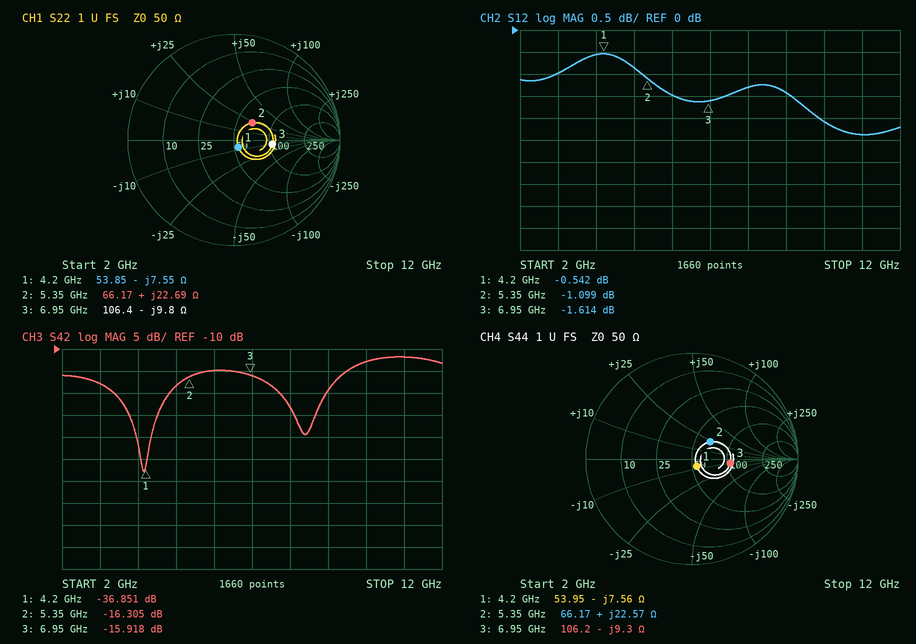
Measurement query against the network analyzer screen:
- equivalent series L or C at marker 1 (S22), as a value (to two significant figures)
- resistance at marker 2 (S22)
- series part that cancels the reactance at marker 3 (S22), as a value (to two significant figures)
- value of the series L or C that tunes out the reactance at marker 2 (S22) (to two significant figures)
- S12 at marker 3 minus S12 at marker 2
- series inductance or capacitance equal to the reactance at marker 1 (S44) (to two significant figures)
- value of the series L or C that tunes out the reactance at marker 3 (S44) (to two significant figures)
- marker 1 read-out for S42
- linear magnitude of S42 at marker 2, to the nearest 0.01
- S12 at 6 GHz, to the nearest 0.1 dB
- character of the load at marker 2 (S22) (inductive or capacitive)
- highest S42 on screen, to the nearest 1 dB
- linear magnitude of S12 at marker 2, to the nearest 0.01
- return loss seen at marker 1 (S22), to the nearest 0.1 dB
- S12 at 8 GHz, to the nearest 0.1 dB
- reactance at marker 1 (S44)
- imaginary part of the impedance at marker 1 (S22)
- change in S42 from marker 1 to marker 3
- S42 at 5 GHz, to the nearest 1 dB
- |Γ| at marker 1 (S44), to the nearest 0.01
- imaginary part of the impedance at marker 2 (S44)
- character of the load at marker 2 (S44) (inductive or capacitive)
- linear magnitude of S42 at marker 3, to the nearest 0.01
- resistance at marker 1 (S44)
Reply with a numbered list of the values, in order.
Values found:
1. 5.0 pF
2. 66.17 Ω
3. 220 pH
4. 1.3 pF
5. -0.515 dB
6. 5.0 pF
7. 210 pH
8. -36.851 dB
9. 0.15
10. -1.5 dB
11. inductive
12. -12 dB
13. 0.88
14. 21.8 dB
15. -1.3 dB
16. -7.56 Ω
17. -7.55 Ω
18. 20.933 dB
19. -18 dB
20. 0.08
21. +22.57 Ω
22. inductive
23. 0.16
24. 53.95 Ω
